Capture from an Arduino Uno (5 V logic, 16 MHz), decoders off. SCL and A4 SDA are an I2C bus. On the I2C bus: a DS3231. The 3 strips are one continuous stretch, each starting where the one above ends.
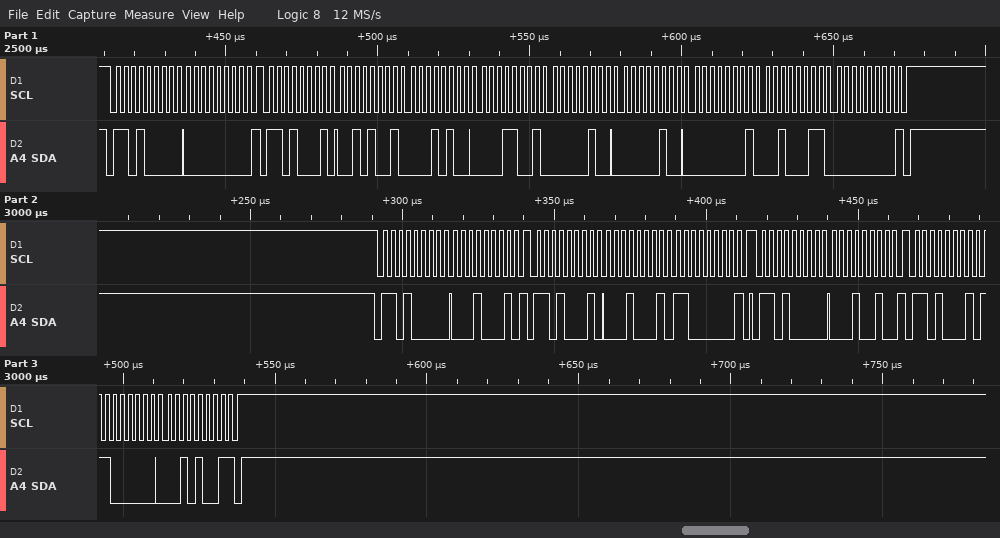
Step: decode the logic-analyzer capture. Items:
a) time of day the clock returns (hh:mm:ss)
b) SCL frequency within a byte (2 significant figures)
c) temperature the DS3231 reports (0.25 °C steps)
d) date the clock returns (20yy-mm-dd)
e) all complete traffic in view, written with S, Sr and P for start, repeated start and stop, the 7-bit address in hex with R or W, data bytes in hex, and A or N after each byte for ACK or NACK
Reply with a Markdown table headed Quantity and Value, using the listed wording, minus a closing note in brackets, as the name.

| Quantity | Value |
|---|---|
| time of day the clock returns | 19:14:29 |
| SCL frequency within a byte | 400 kHz |
| temperature the DS3231 reports | 17.75 °C |
| date the clock returns | 2023-01-04 |
| all complete traffic in view, written with S, Sr and P for start, repeated start and stop, the 7-bit address in hex with R or W, data bytes in hex, and A or N after each byte for ACK or NACK | S 68W A 00 A Sr 68R A 29 A 14 A 19 A 04 A 04 A 01 A 23 A 00 N P S 68W A 11 A Sr 68R A 11 A C0 N P S 68W A 12 A Sr 68R A C0 A 29 N P |
